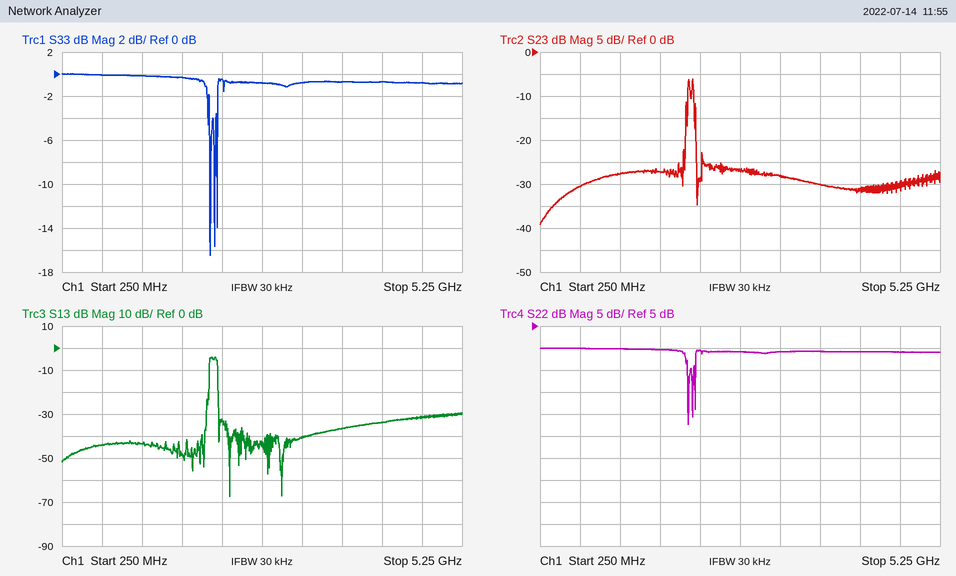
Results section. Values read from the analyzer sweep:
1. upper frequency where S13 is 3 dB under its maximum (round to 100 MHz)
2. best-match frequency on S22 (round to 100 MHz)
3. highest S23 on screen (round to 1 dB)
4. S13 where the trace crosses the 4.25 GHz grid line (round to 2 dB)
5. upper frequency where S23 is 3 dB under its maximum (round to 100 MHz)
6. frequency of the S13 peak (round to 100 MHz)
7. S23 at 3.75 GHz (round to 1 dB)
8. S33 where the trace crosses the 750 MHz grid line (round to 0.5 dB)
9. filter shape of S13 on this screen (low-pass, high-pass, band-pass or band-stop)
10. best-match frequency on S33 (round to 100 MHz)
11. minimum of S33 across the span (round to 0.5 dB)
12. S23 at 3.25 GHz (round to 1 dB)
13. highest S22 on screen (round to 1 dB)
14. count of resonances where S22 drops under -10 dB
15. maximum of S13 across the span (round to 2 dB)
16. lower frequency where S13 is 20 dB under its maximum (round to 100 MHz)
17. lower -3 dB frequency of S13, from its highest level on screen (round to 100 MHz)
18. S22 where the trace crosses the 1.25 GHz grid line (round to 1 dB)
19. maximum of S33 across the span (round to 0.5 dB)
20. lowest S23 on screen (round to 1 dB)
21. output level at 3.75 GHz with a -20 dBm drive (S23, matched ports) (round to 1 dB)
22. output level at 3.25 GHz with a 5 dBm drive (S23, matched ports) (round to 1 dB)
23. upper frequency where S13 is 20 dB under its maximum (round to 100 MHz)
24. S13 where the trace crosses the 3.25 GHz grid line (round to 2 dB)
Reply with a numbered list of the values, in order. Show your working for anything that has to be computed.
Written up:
1. 2.2 GHz
2. 2.1 GHz
3. -6 dB
4. -34 dB
5. 2.2 GHz
6. 2.1 GHz
7. -30 dB
8. 0.0 dB
9. band-pass
10. 2.1 GHz
11. -16.5 dB
12. -28 dB
13. 0 dB
14. 3
15. -4 dB
16. 2.1 GHz
17. 2.1 GHz
18. 0 dB
19. 0.0 dB
20. -39 dB
21. -20 dBm + (-30 dB) = -50 dBm
22. 5 dBm + (-28 dB) = -23 dBm
23. 2.2 GHz
24. -40 dB
